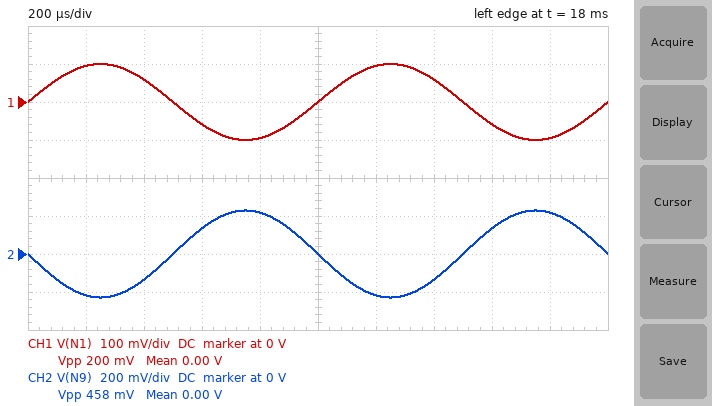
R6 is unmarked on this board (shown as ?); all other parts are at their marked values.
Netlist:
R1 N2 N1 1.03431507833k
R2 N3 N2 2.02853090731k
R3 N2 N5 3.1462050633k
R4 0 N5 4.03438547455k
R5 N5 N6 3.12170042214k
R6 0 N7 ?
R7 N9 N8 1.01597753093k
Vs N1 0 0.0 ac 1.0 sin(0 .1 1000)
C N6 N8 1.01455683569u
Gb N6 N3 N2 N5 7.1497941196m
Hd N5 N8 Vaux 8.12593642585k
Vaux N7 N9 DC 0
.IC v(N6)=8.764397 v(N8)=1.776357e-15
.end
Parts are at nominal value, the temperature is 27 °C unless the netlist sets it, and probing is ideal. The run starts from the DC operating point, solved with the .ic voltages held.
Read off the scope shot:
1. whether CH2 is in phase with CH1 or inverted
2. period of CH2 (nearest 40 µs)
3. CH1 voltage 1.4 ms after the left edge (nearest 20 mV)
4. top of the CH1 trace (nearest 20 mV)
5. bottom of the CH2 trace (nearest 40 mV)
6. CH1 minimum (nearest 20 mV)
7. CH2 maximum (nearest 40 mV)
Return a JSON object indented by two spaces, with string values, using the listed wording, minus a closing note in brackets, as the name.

{
  "whether CH2 is in phase with CH1 or inverted": "inverted",
  "period of CH2": "1.00 ms",
  "CH1 voltage 1.4 ms after the left edge": "60 mV",
  "top of the CH1 trace": "100 mV",
  "bottom of the CH2 trace": "-240 mV",
  "CH1 minimum": "-100 mV",
  "CH2 maximum": "240 mV"
}
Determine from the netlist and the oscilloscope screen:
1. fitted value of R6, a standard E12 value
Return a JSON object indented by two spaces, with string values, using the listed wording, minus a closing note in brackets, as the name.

{
  "fitted value of R6, a standard E12 value": "4.7 kΩ"
}
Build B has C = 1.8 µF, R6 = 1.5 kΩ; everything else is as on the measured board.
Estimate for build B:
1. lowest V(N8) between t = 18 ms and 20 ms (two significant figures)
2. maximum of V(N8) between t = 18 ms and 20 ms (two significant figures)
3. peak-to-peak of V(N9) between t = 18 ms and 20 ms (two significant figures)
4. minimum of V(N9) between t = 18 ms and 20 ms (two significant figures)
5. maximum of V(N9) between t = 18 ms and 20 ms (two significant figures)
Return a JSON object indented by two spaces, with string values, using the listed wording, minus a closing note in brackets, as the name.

{
  "lowest V(N8) between t = 18 ms and 20 ms": "-42 mV",
  "maximum of V(N8) between t = 18 ms and 20 ms": "42 mV",
  "peak-to-peak of V(N9) between t = 18 ms and 20 ms": "50 mV",
  "minimum of V(N9) between t = 18 ms and 20 ms": "-25 mV",
  "maximum of V(N9) between t = 18 ms and 20 ms": "25 mV"
}
